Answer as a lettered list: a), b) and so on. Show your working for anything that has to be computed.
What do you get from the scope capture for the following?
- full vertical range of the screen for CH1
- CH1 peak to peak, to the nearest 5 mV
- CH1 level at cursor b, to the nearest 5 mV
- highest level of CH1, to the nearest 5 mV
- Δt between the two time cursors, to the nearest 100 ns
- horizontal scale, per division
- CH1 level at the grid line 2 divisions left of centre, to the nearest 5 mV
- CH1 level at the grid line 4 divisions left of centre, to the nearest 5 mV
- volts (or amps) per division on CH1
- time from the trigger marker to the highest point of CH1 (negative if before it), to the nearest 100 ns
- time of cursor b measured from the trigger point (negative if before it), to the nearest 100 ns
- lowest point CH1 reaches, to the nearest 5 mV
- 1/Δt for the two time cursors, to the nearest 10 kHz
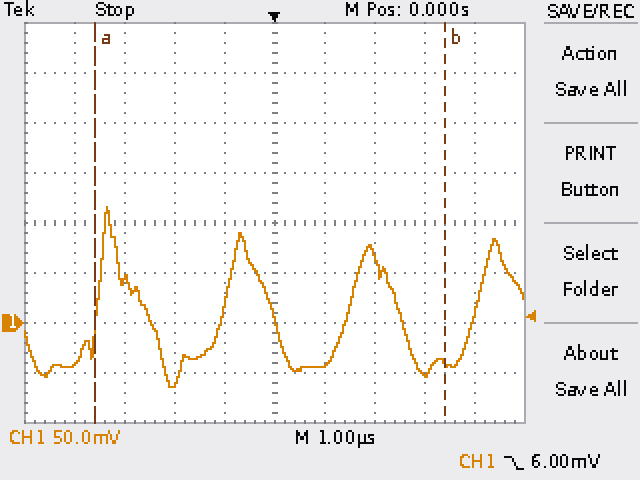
a) 400 mV
b) 115 mV − (-65 mV) = 180 mV
c) -40 mV
d) 115 mV
e) 7.0 µs
f) 1 µs
g) -60 mV
h) -40 mV
i) 50 mV
j) -3.3 µs
k) +3.4 µs
l) -65 mV
m) 1 / 7.0 µs ≈ 140 kHz
